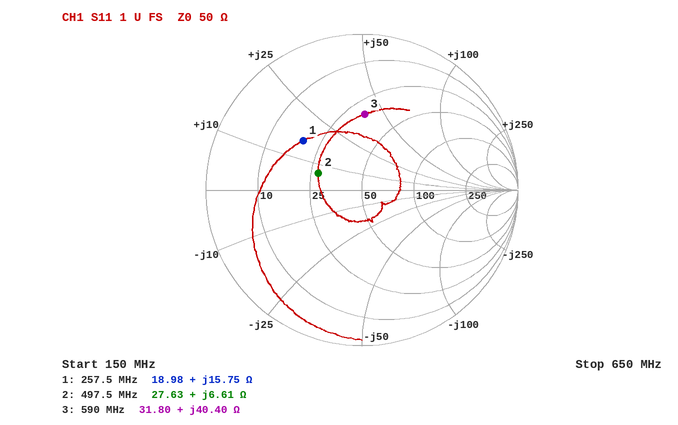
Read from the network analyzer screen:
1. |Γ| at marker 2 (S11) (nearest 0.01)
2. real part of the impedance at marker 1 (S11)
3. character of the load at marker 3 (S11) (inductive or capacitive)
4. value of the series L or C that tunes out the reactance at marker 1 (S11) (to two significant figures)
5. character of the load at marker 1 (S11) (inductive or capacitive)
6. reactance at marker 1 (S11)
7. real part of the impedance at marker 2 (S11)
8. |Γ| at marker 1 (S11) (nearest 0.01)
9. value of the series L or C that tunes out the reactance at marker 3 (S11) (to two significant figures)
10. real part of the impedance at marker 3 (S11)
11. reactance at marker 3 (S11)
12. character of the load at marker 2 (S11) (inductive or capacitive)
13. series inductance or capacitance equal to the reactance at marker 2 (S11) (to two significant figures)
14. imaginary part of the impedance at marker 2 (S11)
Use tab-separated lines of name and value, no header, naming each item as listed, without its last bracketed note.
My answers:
|Γ| at marker 2 (S11)	0.30
real part of the impedance at marker 1	18.98 Ω
character of the load at marker 3 (S11)	inductive
value of the series L or C that tunes out the reactance at marker 1 (S11)	39 pF
character of the load at marker 1 (S11)	inductive
reactance at marker 1	+15.75 Ω
real part of the impedance at marker 2	27.63 Ω
|Γ| at marker 1 (S11)	0.49
value of the series L or C that tunes out the reactance at marker 3 (S11)	6.7 pF
real part of the impedance at marker 3	31.80 Ω
reactance at marker 3	+40.40 Ω
character of the load at marker 2 (S11)	inductive
series inductance or capacitance equal to the reactance at marker 2 (S11)	2.1 nH
imaginary part of the impedance at marker 2	+6.61 Ω
